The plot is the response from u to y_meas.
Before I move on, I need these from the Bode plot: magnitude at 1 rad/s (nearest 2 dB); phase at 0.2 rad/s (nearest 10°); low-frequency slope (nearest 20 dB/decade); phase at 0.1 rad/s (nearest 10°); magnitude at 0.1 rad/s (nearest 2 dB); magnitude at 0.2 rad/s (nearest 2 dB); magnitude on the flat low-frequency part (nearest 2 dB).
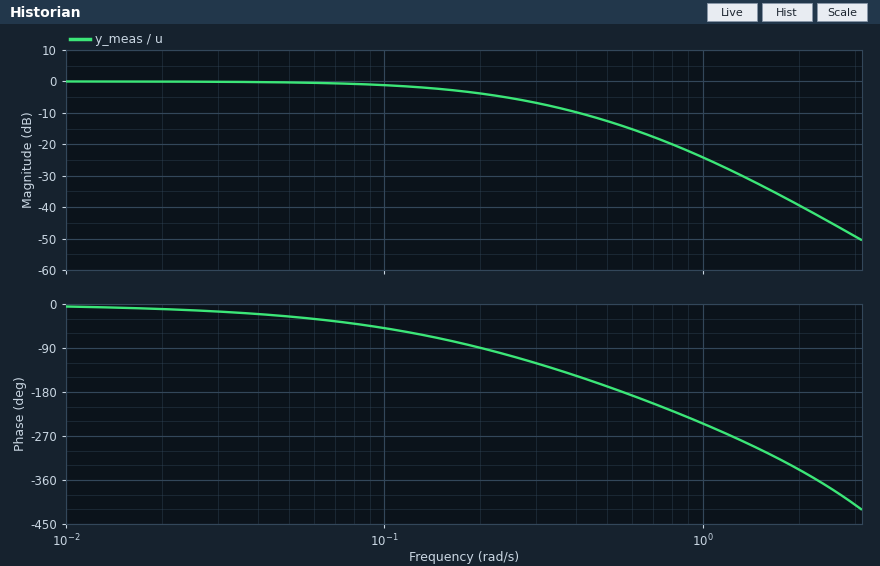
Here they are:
-24 dB
-90°
0 dB/decade
-50°
-2 dB
-4 dB
0 dB
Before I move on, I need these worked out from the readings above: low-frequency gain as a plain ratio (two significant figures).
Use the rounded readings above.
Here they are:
1.0
